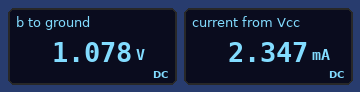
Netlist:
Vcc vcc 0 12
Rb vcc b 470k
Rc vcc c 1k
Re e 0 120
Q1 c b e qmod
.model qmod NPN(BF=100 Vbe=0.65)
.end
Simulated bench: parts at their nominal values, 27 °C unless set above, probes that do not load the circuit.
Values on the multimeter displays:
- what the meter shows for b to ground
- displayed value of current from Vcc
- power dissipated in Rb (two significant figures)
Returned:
1.078 V
2.347 mA
250 µW
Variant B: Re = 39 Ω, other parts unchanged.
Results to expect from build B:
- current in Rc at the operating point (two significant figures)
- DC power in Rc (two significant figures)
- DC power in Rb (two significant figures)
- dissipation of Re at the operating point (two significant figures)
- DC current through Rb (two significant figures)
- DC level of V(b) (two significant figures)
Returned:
2.4 mA
5.6 mW
260 µW
220 µW
24 µA
890 mV
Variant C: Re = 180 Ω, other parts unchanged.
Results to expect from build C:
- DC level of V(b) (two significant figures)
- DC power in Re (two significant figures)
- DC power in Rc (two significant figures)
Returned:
1.2 V
970 µW
5.3 mW
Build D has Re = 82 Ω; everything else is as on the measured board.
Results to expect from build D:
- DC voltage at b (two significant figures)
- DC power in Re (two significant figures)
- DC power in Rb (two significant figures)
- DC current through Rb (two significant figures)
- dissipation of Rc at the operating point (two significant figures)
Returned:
990 mV
460 µW
260 µW
23 µA
5.5 mW
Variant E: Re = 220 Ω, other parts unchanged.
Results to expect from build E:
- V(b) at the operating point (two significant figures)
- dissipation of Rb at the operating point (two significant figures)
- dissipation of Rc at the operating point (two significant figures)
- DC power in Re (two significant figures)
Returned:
1.3 V
240 µW
5.2 mW
1.2 mW
